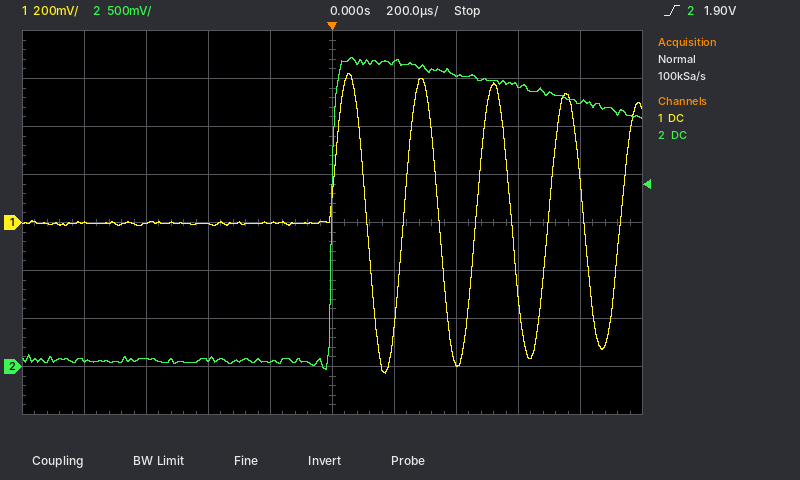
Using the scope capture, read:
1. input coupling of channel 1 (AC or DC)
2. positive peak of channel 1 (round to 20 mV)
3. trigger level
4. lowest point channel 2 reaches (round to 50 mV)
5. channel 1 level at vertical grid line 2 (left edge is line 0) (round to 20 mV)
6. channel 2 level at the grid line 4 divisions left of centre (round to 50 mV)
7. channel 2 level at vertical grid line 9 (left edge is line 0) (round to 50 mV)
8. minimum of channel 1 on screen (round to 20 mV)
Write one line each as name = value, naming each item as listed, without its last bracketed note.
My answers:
input coupling of channel 1 = DC
positive peak of channel 1 = 620 mV
trigger level = 1.90 V
lowest point channel 2 reaches = -50 mV
channel 1 level at vertical grid line 2 (left edge is line 0) = 0 mV
channel 2 level at the grid line 4 divisions left of centre = 50 mV
channel 2 level at vertical grid line 9 (left edge is line 0) = 2.75 V
minimum of channel 1 on screen = -620 mV
